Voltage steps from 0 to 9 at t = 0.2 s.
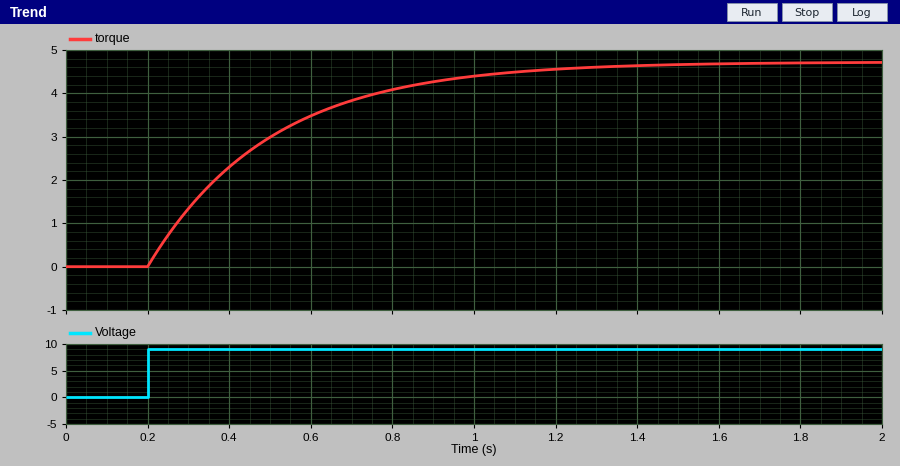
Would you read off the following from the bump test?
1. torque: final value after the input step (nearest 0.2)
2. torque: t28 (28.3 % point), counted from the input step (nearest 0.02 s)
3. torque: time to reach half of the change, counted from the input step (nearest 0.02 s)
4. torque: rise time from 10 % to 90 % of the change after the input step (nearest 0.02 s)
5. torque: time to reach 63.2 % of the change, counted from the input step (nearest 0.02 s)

4.8
0.10 s
0.20 s
0.66 s
0.30 s
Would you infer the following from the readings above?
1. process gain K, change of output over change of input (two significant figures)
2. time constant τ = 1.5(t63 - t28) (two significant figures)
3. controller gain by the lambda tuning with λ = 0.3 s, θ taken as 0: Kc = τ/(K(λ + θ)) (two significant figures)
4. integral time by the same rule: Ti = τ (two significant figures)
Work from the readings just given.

0.53
0.30 s
1.9
0.30 s
